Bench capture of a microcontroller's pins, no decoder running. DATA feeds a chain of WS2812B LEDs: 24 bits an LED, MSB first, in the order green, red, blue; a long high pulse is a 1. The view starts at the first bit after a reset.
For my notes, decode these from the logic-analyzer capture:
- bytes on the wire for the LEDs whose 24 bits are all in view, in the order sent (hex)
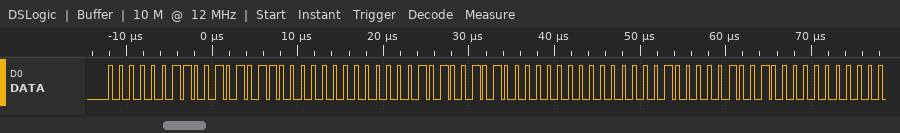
03 2B 00 05 28 00 08 24 00
